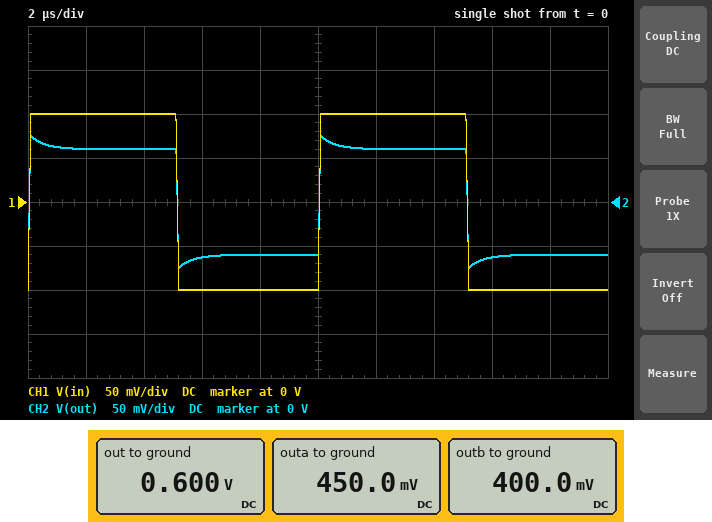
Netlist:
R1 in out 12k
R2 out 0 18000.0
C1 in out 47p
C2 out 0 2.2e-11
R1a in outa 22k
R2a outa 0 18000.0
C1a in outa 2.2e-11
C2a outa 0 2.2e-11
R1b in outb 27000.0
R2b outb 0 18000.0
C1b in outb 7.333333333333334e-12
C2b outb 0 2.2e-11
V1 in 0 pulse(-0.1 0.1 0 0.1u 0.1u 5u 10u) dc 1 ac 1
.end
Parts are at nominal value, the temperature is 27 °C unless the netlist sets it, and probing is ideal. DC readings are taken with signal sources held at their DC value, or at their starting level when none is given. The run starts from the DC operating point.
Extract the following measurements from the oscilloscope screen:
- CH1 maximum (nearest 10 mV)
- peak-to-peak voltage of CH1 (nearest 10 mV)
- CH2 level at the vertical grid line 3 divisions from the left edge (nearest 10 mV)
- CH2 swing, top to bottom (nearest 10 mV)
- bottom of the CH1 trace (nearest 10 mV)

100 mV
200 mV
-60 mV
150 mV
-100 mV
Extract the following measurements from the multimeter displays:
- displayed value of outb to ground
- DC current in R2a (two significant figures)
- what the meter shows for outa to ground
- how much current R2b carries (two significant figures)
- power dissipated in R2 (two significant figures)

400.0 mV
25 µA
450.0 mV
22 µA
20 µW
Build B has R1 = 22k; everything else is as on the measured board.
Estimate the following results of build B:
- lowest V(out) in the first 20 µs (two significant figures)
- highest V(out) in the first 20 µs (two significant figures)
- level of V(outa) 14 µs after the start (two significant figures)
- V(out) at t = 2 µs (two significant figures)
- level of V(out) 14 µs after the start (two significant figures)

-88 mV
88 mV
45 mV
48 mV
45 mV
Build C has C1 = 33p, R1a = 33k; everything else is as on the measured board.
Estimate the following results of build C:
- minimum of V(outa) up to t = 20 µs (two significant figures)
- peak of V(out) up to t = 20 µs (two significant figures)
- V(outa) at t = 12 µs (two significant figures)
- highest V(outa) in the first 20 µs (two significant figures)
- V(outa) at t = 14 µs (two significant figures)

-62 mV
60 mV
36 mV
62 mV
35 mV
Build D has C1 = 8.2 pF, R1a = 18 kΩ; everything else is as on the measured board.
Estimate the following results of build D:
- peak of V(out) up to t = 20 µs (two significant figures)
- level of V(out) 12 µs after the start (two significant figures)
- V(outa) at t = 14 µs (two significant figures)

60 mV
60 mV
50 mV
